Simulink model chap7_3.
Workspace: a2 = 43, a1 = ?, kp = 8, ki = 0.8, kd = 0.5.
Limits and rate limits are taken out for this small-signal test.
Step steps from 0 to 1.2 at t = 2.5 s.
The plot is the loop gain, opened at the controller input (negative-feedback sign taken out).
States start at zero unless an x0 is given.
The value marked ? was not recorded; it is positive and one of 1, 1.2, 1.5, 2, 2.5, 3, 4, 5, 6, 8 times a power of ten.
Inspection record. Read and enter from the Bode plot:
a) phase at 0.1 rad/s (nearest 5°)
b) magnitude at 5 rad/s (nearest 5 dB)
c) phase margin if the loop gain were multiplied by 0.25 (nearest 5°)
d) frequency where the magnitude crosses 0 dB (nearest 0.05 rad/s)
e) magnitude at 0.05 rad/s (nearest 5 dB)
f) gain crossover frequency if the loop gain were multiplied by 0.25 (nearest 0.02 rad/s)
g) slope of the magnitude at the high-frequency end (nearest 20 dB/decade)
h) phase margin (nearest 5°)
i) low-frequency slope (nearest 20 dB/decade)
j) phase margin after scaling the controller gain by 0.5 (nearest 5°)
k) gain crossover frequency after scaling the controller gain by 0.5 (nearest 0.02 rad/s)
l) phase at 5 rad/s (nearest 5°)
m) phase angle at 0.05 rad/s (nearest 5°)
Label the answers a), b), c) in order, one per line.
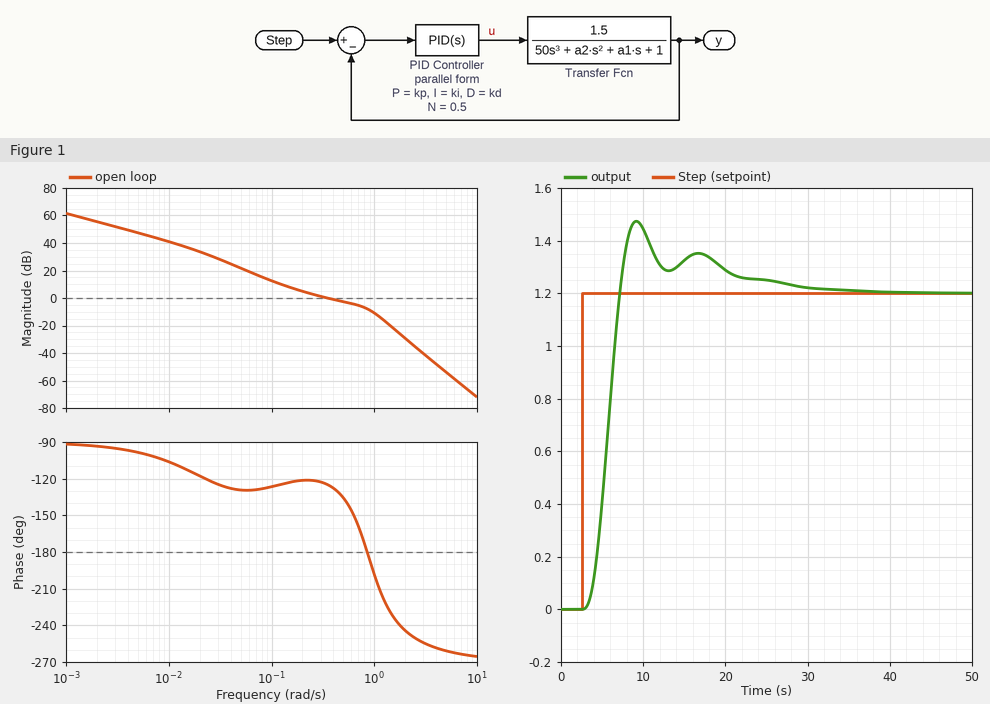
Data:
a) -125°
b) -55 dB
c) 55°
d) 0.35 rad/s
e) 20 dB
f) 0.10 rad/s
g) -60 dB/decade
h) 55°
i) -20 dB/decade
j) 60°
k) 0.18 rad/s
l) -260°
m) -130°
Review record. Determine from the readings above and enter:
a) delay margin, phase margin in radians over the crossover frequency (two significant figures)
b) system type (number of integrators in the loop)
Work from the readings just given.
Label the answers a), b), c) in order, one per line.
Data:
a) 2.7 s
b) 1
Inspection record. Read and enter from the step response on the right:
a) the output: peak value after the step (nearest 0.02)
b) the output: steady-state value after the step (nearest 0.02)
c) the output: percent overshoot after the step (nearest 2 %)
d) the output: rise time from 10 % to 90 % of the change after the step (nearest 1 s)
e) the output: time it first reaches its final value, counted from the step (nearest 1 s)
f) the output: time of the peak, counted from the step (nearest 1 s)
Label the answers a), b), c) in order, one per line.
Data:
a) 1.48
b) 1.20
c) 22 %
d) 3 s
e) 5 s
f) 7 s
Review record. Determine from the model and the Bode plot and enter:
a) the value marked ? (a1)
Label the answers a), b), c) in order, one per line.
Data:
a) 40
